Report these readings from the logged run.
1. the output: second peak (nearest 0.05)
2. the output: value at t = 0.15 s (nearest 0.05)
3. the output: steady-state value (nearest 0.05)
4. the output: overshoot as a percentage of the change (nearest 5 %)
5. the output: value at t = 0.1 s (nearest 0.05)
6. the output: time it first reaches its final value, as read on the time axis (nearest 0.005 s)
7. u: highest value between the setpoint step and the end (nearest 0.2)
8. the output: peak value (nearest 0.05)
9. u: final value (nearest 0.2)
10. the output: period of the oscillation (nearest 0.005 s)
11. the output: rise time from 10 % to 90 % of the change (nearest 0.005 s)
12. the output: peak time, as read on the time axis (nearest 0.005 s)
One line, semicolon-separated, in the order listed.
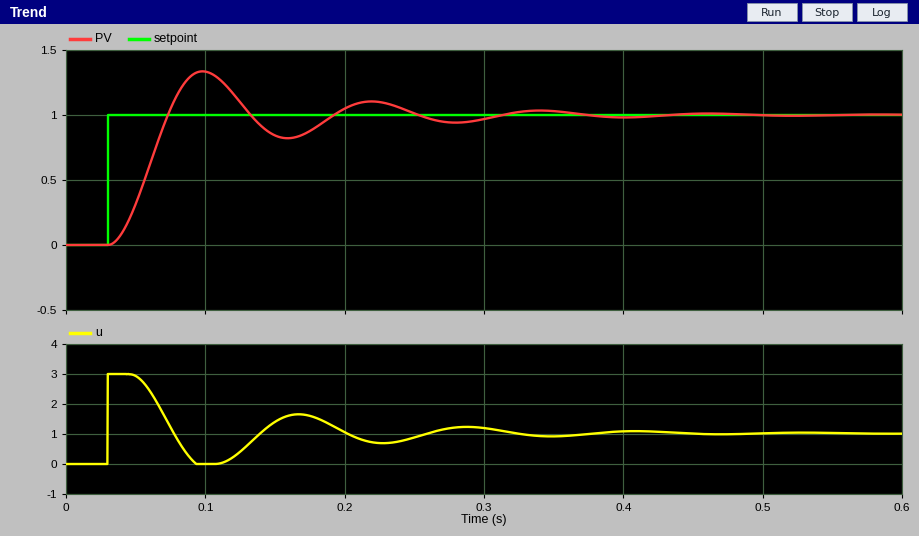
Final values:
1.10; 0.85; 1.00; 35 %; 1.35; 0.075 s; 3.0; 1.35; 1.0; 0.120 s; 0.030 s; 0.100 s
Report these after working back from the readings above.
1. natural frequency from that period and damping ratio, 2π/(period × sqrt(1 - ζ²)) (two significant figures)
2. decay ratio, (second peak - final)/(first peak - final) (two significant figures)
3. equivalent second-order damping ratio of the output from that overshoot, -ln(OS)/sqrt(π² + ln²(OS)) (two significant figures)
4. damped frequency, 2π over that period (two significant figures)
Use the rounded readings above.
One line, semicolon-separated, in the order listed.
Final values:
55 rad/s; 0.29; 0.32; 52 rad/s
